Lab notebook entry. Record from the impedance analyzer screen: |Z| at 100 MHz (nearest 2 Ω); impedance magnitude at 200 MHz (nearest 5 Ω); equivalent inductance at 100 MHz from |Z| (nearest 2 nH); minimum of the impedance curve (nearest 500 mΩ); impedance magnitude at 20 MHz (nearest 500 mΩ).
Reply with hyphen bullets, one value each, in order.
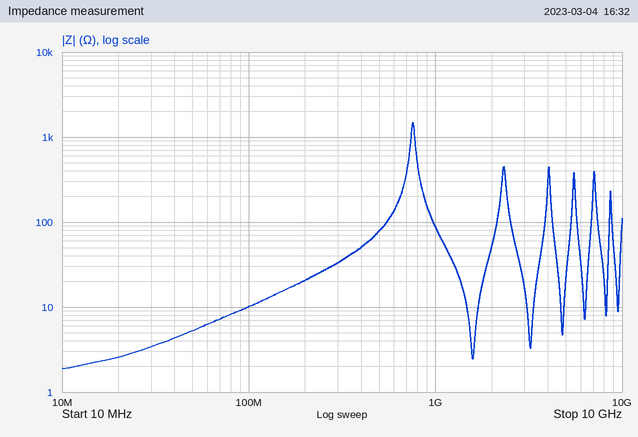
- 10 Ω
- 20 Ω
- 16 nH
- 2.0 Ω
- 2.5 Ω
